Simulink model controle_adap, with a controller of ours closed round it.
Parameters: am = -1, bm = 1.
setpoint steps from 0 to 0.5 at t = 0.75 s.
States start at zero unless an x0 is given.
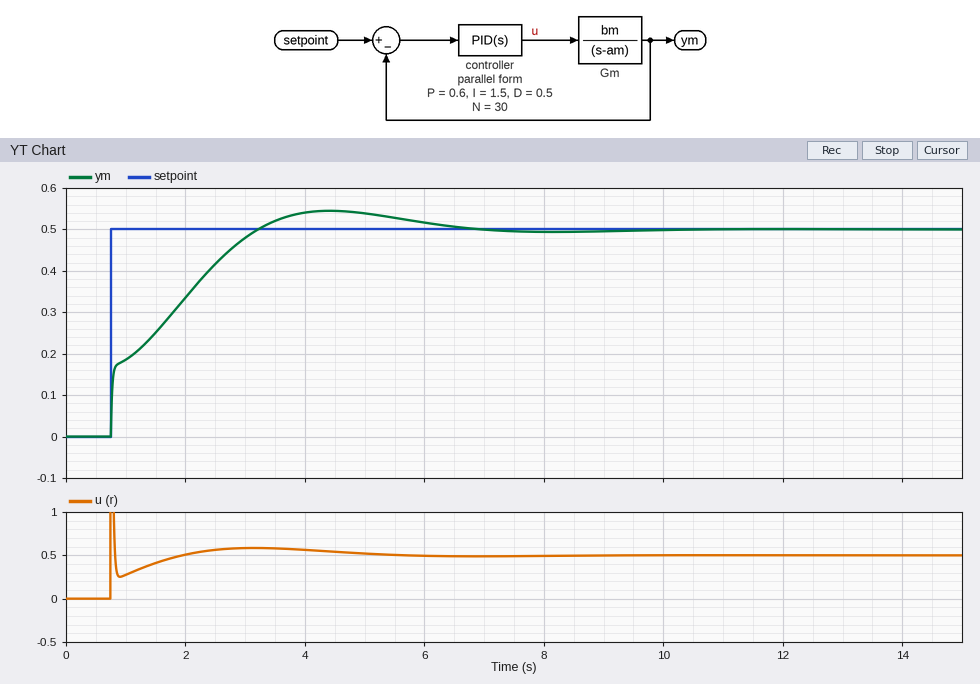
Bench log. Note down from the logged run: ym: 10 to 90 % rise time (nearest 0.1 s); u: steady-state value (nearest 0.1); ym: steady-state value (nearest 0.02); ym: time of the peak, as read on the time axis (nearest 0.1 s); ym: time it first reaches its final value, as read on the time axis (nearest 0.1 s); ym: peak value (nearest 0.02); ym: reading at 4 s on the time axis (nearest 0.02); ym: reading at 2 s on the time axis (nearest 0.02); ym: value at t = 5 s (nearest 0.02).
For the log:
2.0 s
0.5
0.50
4.4 s
3.2 s
0.54
0.54
0.34
0.54
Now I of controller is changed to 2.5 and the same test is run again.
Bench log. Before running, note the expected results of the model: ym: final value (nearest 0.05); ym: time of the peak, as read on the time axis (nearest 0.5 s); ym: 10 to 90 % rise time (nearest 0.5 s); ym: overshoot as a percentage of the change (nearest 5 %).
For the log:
0.50
3.5 s
1.5 s
15 %
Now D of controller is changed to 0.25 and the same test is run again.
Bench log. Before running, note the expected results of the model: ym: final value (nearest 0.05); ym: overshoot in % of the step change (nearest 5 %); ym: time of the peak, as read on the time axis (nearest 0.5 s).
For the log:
0.50
10 %
4.0 s
